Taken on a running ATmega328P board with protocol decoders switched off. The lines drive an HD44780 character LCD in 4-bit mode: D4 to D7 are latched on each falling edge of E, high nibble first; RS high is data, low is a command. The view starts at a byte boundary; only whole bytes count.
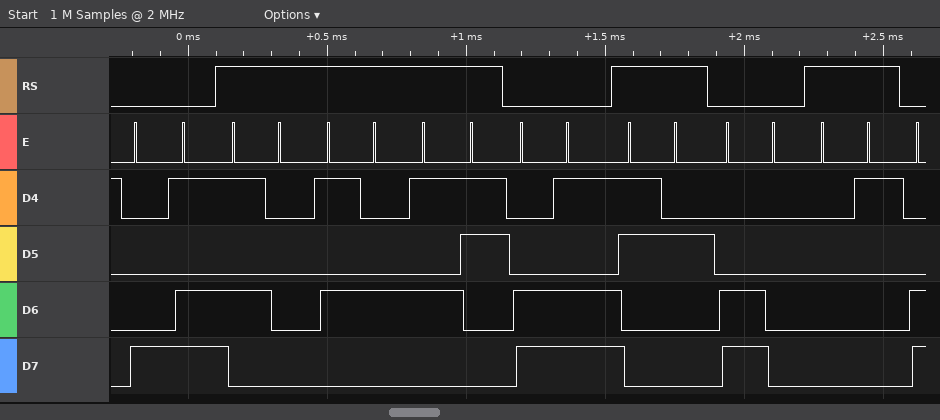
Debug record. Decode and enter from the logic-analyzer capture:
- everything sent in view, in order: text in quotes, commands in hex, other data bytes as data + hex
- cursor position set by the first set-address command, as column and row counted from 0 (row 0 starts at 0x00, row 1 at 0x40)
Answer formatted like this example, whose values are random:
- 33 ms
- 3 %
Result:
- 0x8D "PTS" 0xCD "2" 0xC0 data 01
- column 13, row 0
